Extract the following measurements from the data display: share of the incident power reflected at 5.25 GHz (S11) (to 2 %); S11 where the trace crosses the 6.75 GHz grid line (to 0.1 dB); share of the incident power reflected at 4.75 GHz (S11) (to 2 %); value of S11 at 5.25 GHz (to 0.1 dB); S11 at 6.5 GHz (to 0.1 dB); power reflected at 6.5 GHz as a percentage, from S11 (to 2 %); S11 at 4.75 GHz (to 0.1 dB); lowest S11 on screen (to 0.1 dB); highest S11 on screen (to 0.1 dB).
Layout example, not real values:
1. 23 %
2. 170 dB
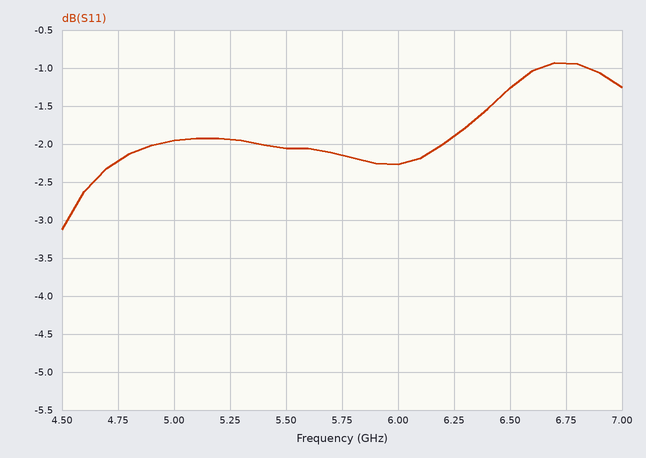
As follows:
1. 64 %
2. -0.9 dB
3. 60 %
4. -1.9 dB
5. -1.3 dB
6. 74 %
7. -2.2 dB
8. -3.1 dB
9. -0.9 dB
